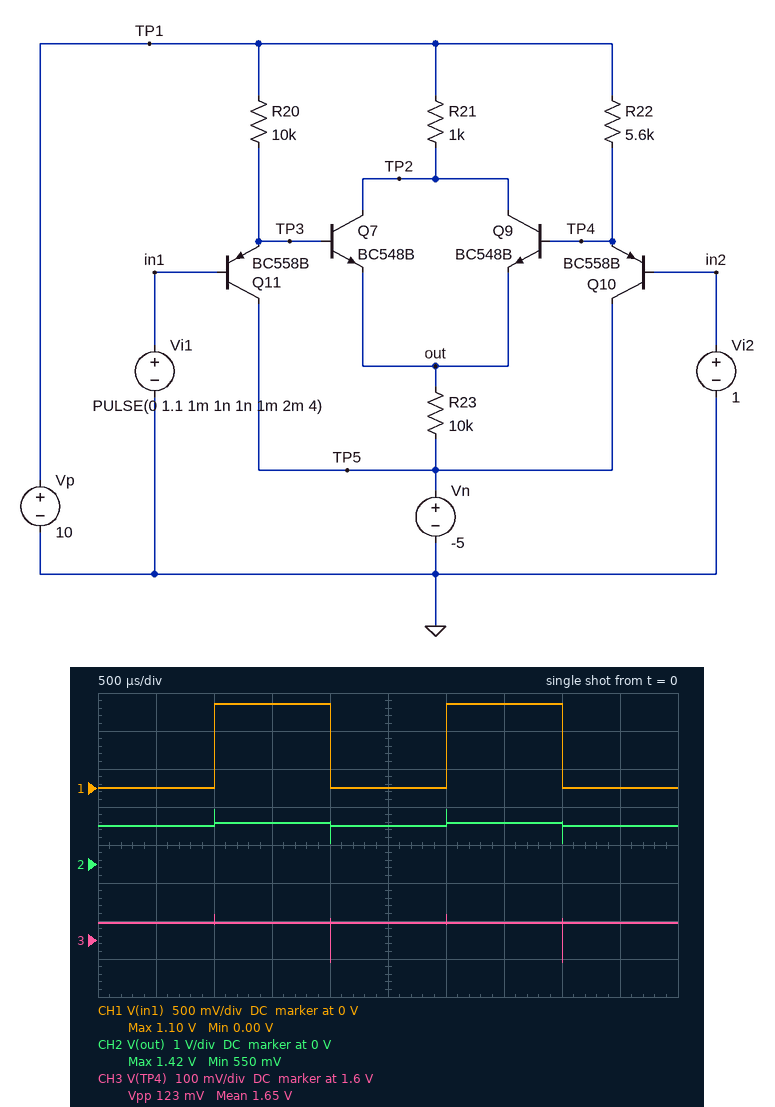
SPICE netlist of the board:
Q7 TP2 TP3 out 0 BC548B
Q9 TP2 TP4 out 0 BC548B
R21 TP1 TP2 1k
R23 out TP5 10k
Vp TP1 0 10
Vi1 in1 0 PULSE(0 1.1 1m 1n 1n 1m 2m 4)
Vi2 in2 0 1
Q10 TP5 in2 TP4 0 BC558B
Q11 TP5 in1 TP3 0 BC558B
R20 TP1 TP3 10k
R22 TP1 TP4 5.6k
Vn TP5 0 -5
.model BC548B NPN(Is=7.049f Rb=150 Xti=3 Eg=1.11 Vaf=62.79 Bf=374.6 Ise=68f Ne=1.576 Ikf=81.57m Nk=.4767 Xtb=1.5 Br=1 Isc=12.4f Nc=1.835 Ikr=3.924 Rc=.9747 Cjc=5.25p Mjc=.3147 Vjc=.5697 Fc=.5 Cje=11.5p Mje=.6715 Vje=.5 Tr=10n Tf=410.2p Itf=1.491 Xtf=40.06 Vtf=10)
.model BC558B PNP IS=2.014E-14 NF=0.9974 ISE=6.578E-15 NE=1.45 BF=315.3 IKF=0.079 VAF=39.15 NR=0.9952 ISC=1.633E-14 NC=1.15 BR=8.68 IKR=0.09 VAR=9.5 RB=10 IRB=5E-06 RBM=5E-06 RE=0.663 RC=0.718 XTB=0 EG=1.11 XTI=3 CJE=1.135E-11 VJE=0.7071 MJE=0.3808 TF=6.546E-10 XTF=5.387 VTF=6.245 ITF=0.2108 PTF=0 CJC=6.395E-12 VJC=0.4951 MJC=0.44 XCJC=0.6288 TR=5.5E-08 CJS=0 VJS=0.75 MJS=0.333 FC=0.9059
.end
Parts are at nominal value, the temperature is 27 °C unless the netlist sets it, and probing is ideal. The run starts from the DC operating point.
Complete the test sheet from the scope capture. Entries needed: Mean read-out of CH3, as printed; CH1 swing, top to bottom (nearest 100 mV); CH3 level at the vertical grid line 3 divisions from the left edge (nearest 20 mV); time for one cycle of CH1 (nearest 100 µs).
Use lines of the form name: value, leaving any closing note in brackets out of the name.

Mean read-out of CH3, as printed: 1.65 V
CH1 swing, top to bottom: 1.1 V
CH3 level at the vertical grid line 3 divisions from the left edge: 1.64 V
time for one cycle of CH1: 2.0 ms
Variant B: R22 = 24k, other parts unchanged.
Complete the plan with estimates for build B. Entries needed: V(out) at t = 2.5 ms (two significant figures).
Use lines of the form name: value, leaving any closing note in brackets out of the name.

V(out) at t = 2.5 ms: 960 mV
